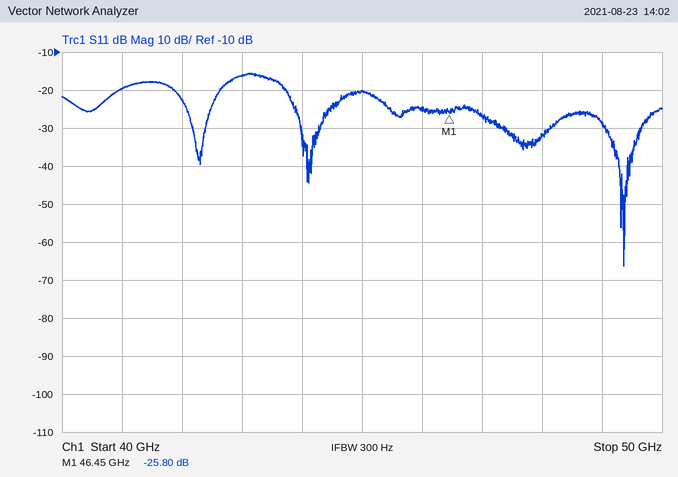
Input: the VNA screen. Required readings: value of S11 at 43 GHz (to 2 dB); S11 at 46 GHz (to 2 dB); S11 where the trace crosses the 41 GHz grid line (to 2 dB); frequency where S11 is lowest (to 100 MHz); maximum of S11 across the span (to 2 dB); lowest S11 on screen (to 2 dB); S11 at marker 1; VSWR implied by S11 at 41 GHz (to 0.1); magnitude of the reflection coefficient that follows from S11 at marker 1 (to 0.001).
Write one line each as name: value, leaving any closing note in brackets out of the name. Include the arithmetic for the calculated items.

value of S11 at 43 GHz: -16 dB
S11 at 46 GHz: -24 dB
S11 where the trace crosses the 41 GHz grid line: -20 dB
frequency where S11 is lowest: 49.4 GHz
maximum of S11 across the span: -16 dB
lowest S11 on screen: -66 dB
S11 at marker 1: -25.80 dB
VSWR implied by S11 at 41 GHz: |Γ| = 10^(-20/20) = 0.1000; VSWR = (1 + 0.1000)/(1 − 0.1000) ≈ 1.2
magnitude of the reflection coefficient that follows from S11 at marker 1: 10^(-25.8/20) ≈ 0.051
